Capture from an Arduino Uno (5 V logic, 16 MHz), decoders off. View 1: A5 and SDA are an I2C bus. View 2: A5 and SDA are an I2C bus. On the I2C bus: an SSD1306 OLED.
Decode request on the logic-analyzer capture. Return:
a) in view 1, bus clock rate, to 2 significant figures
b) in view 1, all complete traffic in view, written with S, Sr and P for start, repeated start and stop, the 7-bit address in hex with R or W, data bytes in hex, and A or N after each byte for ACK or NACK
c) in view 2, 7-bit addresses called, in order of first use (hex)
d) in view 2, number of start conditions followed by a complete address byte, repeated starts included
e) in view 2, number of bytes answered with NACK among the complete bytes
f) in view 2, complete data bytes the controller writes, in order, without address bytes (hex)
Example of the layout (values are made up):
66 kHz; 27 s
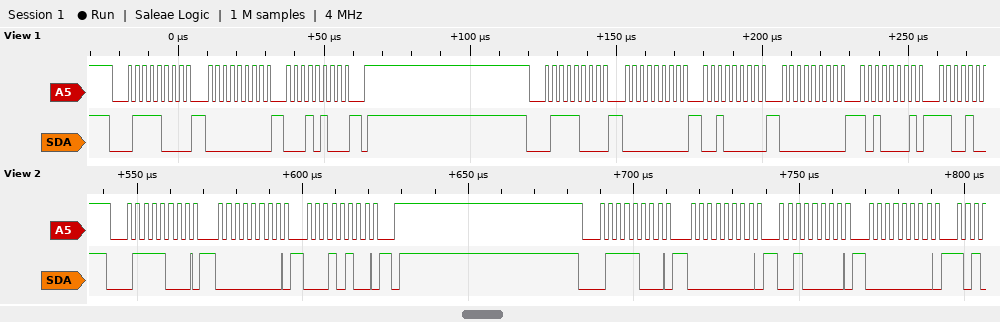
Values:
400 kHz; S 3CW A 00 A 14 A P S 3CW A 00 A 20 A 00 A A1 A; 0x3C; 2; 0; 00 14 00 20 00
